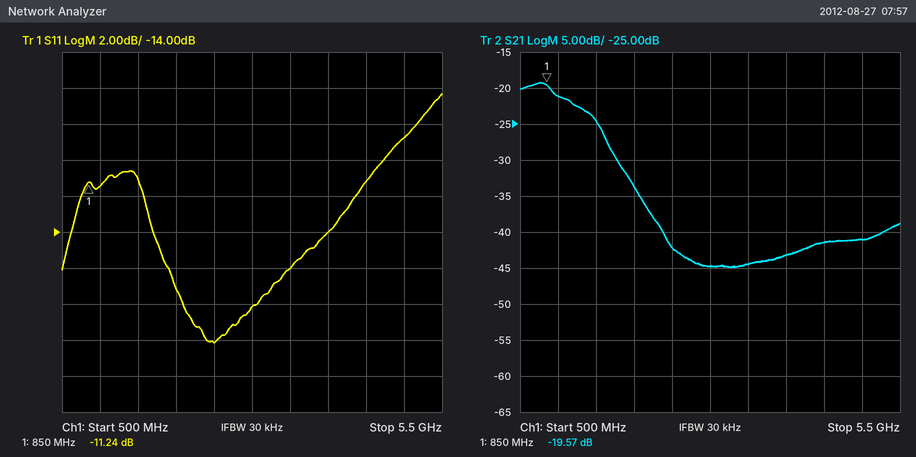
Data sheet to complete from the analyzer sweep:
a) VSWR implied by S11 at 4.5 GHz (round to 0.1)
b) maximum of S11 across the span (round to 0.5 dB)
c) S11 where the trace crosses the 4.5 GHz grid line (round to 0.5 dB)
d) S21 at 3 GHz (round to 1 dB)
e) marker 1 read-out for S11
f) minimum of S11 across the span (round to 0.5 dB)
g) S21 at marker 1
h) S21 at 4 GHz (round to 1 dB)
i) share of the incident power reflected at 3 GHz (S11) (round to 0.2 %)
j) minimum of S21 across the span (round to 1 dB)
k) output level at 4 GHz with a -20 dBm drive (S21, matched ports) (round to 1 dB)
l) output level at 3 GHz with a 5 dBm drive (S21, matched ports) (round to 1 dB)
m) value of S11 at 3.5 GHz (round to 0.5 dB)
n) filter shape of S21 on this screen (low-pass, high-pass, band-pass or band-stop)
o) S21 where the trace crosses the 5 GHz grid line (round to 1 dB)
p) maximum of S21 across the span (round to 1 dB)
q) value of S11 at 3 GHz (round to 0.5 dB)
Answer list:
1.8
-6.5 dB
-11.0 dB
-45 dB
-11.24 dB
-20.0 dB
-19.57 dB
-43 dB
1.6 %
-45 dB
-63 dBm
-40 dBm
-16.0 dB
low-pass
-41 dB
-19 dB
-18.0 dB
